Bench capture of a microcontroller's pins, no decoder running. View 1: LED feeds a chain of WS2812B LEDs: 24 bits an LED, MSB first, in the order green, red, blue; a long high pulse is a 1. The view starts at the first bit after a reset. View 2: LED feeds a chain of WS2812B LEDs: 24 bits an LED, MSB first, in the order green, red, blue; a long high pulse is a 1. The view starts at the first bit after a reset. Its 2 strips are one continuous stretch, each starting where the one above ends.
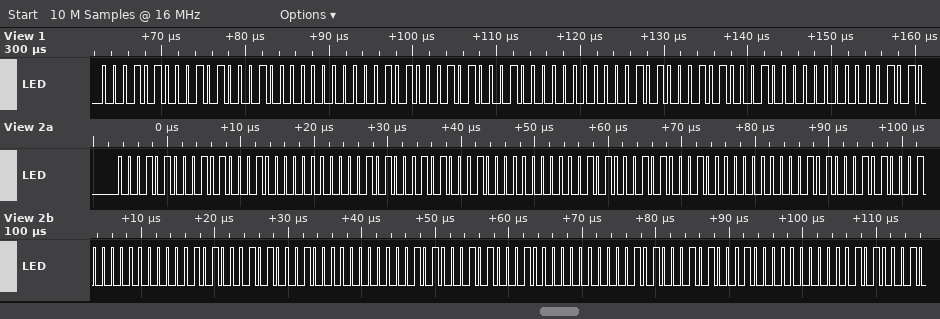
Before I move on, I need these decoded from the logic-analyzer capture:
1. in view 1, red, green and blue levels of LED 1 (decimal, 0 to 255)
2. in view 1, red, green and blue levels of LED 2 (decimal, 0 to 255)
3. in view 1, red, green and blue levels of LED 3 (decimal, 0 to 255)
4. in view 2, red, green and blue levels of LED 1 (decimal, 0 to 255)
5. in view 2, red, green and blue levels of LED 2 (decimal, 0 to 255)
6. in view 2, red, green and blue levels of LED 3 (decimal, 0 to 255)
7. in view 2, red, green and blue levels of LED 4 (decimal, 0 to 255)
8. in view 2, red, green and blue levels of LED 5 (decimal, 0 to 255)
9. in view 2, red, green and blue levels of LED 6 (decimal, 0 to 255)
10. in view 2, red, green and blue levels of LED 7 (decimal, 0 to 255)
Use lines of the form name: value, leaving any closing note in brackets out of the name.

in view 1, red, green and blue levels of LED 1: 81, 20, 0
in view 1, red, green and blue levels of LED 2: 81, 20, 0
in view 1, red, green and blue levels of LED 3: 81, 20, 0
in view 2, red, green and blue levels of LED 1: 81, 20, 0
in view 2, red, green and blue levels of LED 2: 81, 20, 0
in view 2, red, green and blue levels of LED 3: 81, 20, 0
in view 2, red, green and blue levels of LED 4: 81, 20, 0
in view 2, red, green and blue levels of LED 5: 81, 20, 0
in view 2, red, green and blue levels of LED 6: 81, 20, 0
in view 2, red, green and blue levels of LED 7: 81, 20, 0
